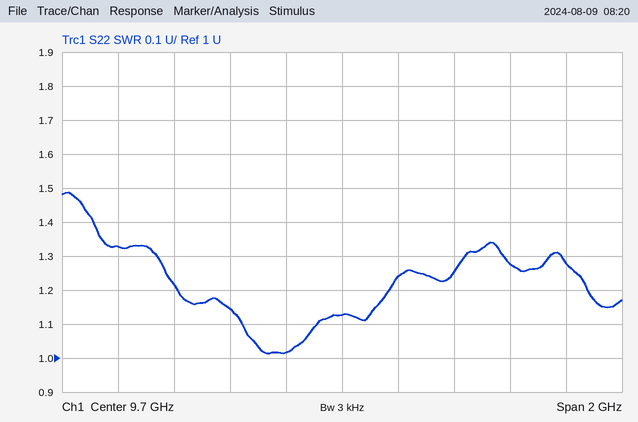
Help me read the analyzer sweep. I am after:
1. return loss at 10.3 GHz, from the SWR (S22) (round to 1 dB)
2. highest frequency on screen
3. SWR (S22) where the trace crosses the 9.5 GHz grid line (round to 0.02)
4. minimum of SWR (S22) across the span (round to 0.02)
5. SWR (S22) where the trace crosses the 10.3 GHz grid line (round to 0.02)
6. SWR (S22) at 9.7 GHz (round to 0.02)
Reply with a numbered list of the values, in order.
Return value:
1. 18 dB
2. 10.7 GHz
3. 1.02
4. 1.02
5. 1.28
6. 1.12
